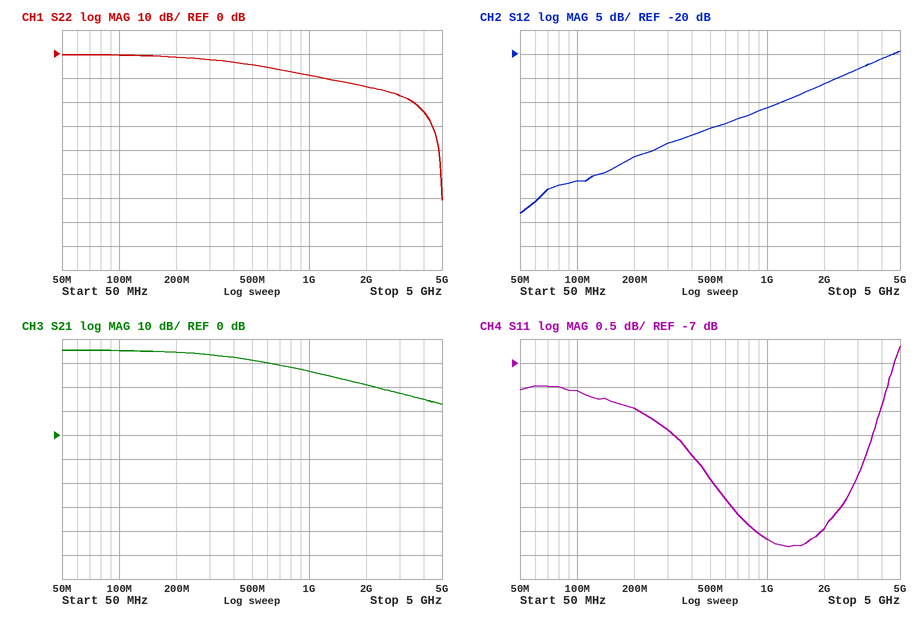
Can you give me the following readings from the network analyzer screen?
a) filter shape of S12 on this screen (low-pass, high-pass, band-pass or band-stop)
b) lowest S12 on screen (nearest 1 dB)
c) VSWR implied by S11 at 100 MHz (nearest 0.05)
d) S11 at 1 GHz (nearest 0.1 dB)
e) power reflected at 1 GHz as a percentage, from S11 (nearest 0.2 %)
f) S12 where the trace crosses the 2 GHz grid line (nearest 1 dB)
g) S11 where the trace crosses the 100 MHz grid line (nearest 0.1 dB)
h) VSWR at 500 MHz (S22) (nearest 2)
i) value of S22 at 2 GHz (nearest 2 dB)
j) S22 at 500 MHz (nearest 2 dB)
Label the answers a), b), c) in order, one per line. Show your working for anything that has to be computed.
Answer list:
a) high-pass
b) -53 dB
c) |Γ| = 10^(-7.6/20) = 0.4169; VSWR = (1 + 0.4169)/(1 − 0.4169) ≈ 2.43, so 2.45 to the nearest 0.05
d) -10.7 dB
e) 10^(-10.7/10) ≈ 8.51 %, so 8.6 % to the nearest 0.2 %
f) -26 dB
g) -7.6 dB
h) |Γ| = 10^(-4/20) = 0.6310; VSWR = (1 + 0.6310)/(1 − 0.6310) ≈ 4
i) -14 dB
j) -4 dB
